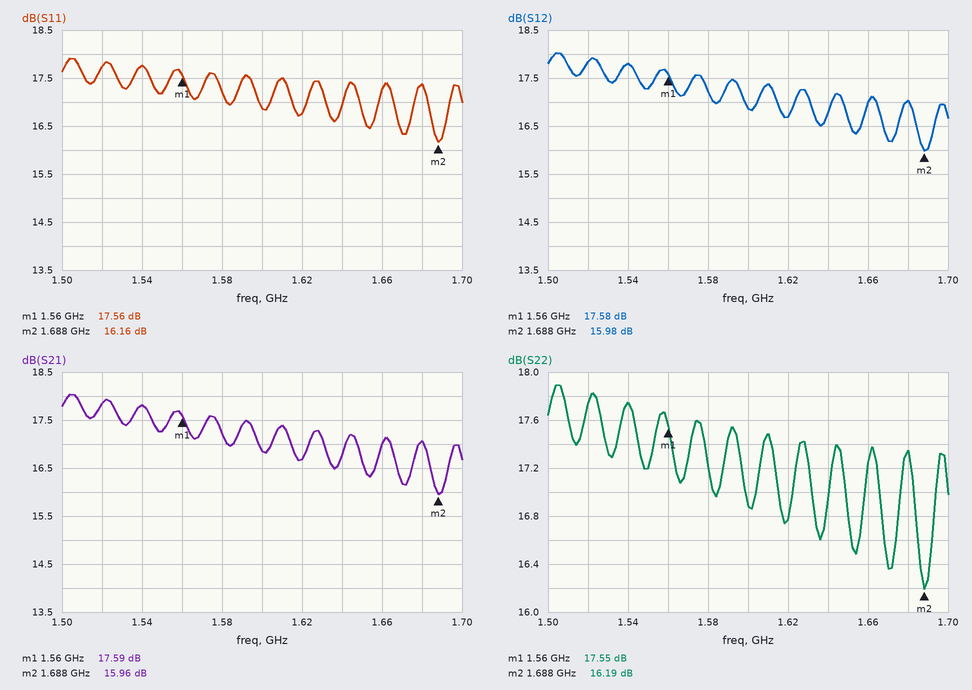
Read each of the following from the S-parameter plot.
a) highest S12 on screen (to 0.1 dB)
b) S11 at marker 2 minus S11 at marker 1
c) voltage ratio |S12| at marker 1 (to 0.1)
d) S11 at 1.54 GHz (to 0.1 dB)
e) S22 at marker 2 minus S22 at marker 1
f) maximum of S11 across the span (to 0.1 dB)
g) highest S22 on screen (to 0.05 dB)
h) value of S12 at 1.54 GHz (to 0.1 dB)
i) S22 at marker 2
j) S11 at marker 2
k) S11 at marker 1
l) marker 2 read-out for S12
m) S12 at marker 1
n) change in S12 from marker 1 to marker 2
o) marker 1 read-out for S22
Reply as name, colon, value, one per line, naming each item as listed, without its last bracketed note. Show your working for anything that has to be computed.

highest S12 on screen: 18.0 dB
S11 at marker 2 minus S11 at marker 1: 16.16 − (17.56) = -1.40 dB
voltage ratio |S12| at marker 1: 10^(17.58/20) ≈ 7.6
S11 at 1.54 GHz: 17.8 dB
S22 at marker 2 minus S22 at marker 1: 16.19 − (17.55) = -1.36 dB
maximum of S11 across the span: 17.9 dB
highest S22 on screen: 17.90 dB
value of S12 at 1.54 GHz: 17.8 dB
S22 at marker 2: 16.19 dB
S11 at marker 2: 16.16 dB
S11 at marker 1: 17.56 dB
marker 2 read-out for S12: 15.98 dB
S12 at marker 1: 17.58 dB
change in S12 from marker 1 to marker 2: 15.98 − (17.58) = -1.60 dB
marker 1 read-out for S22: 17.55 dB
